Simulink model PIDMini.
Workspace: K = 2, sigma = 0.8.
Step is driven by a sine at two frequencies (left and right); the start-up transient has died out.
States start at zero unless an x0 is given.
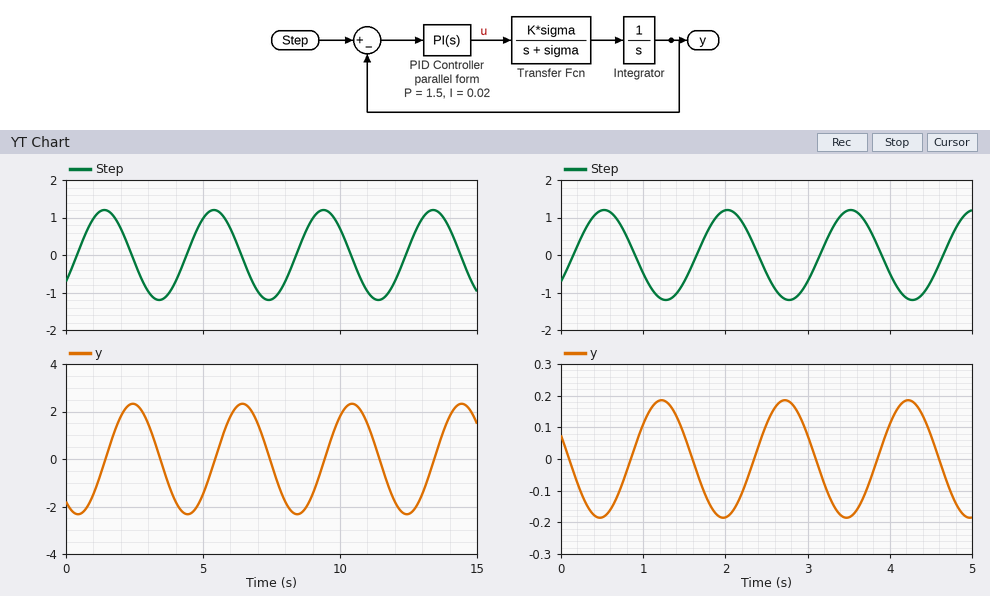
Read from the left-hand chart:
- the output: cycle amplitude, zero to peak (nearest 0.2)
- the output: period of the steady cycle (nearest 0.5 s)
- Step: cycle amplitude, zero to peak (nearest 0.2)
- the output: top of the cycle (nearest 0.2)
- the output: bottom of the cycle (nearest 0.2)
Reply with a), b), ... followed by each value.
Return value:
a) 2.4
b) 4.0 s
c) 1.2
d) 2.4
e) -2.4
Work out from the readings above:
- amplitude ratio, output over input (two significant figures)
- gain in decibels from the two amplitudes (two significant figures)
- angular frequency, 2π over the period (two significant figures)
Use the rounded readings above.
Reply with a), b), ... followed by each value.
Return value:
a) 2.0
b) 6.0 dB
c) 1.6 rad/s
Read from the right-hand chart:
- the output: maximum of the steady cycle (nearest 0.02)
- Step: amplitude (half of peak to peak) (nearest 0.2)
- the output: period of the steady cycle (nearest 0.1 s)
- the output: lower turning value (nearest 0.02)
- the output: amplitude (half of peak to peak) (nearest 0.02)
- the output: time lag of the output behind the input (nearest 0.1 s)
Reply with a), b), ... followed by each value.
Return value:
a) 0.18
b) 1.2
c) 1.5 s
d) -0.18
e) 0.18
f) 0.7 s
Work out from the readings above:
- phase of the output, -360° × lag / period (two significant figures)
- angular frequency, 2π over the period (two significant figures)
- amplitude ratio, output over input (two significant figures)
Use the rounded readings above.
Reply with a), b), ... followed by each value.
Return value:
a) -170°
b) 4.2 rad/s
c) 0.15
